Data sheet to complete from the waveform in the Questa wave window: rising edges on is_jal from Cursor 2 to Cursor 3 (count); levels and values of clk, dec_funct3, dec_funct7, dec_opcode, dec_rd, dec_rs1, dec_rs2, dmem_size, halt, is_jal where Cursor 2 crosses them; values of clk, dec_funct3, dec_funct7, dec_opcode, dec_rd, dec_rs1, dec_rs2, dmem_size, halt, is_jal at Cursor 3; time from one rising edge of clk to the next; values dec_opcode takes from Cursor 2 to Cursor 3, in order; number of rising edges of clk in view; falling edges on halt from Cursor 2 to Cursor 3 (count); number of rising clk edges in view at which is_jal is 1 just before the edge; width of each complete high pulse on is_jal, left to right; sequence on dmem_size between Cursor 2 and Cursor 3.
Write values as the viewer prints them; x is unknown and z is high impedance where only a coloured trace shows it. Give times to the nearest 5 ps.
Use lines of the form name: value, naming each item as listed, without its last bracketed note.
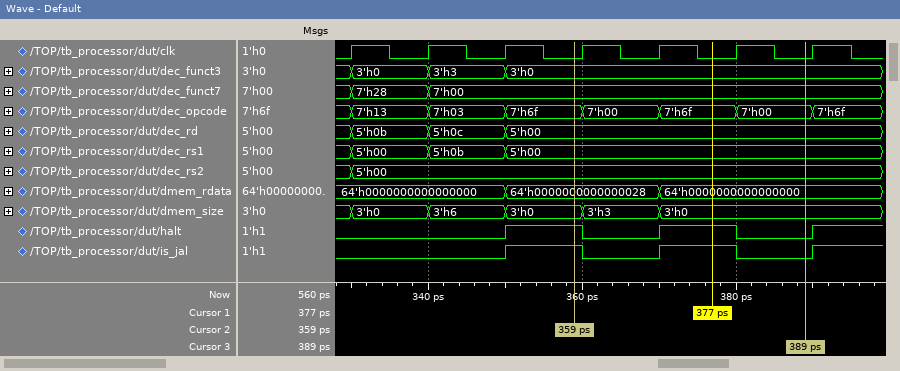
rising edges on is_jal from Cursor 2 to Cursor 3: 1
levels and values of clk, dec_funct3, dec_funct7, dec_opcode, dec_rd, dec_rs1, dec_rs2, dmem_size, halt, is_jal where Cursor 2 crosses them: clk=0, dec_funct3=3'h0, dec_funct7=7'h00, dec_opcode=7'h6f, dec_rd=5'h00, dec_rs1=5'h00, dec_rs2=5'h00, dmem_size=3'h0, halt=1, is_jal=1
values of clk, dec_funct3, dec_funct7, dec_opcode, dec_rd, dec_rs1, dec_rs2, dmem_size, halt, is_jal at Cursor 3: clk=0, dec_funct3=3'h0, dec_funct7=7'h00, dec_opcode=7'h00, dec_rd=5'h00, dec_rs1=5'h00, dec_rs2=5'h00, dmem_size=3'h0, halt=0, is_jal=0
time from one rising edge of clk to the next: 10 ps
values dec_opcode takes from Cursor 2 to Cursor 3, in order: 7'h6f, 7'h00, 7'h6f, 7'h00
number of rising edges of clk in view: 7
falling edges on halt from Cursor 2 to Cursor 3: 2
number of rising clk edges in view at which is_jal is 1 just before the edge: 2
width of each complete high pulse on is_jal, left to right: 10 ps, 10 ps
sequence on dmem_size between Cursor 2 and Cursor 3: 3'h0, 3'h3, 3'h0
